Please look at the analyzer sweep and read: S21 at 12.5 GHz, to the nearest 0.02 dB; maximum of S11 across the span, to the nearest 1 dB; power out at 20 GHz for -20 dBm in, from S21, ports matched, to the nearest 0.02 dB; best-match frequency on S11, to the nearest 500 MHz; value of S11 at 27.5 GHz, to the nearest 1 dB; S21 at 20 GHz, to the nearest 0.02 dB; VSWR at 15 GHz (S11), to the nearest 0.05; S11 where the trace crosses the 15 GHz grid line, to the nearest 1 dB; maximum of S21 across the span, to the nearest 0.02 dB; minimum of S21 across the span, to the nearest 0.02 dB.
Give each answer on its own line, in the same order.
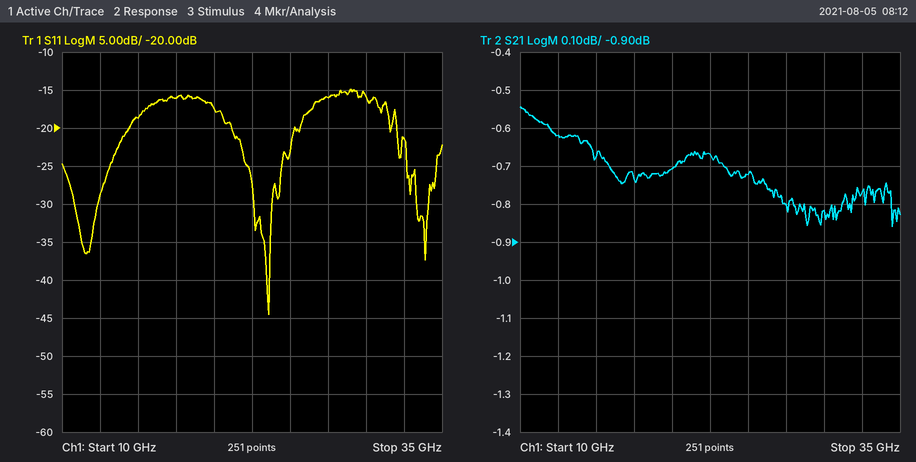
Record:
-0.62 dB
-15 dB
-20.70 dBm
23.5 GHz
-16 dB
-0.70 dB
1.25
-19 dB
-0.54 dB
-0.86 dB
